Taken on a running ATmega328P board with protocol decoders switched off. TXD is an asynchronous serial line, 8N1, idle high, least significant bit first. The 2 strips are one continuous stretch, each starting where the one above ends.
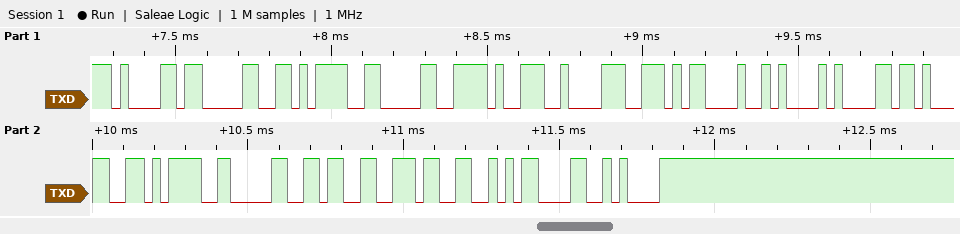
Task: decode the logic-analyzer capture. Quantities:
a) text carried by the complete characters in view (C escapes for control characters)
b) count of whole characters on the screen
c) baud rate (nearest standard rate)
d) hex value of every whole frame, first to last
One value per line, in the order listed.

"a0=098\r\na1=033\r\n"
16
38400 baud
61 30 3D 30 39 38 0D 0A 61 31 3D 30 33 33 0D 0A
